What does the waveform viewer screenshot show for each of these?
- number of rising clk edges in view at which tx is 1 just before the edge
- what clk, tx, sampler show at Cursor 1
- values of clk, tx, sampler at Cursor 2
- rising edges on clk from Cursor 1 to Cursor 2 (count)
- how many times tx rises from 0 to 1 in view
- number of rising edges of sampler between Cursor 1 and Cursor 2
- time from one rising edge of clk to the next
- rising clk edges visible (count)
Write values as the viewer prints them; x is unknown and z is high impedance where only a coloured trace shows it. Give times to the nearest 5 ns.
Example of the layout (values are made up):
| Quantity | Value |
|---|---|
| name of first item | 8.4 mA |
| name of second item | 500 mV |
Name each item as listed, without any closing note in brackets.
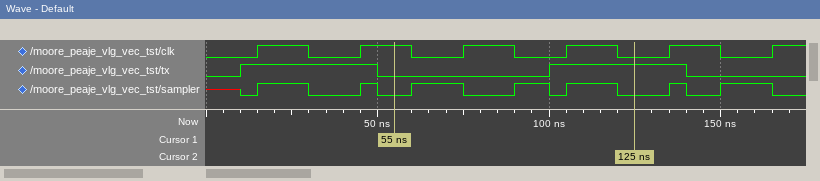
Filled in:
| Quantity | Value |
|---|---|
| number of rising clk edges in view at which tx is 1 just before the edge | 4 |
| what clk, tx, sampler show at Cursor 1 | clk=1, tx=0, sampler=0 |
| values of clk, tx, sampler at Cursor 2 | clk=0, tx=1, sampler=0 |
| rising edges on clk from Cursor 1 to Cursor 2 | 2 |
| how many times tx rises from 0 to 1 in view | 2 |
| number of rising edges of sampler between Cursor 1 and Cursor 2 | 3 |
| time from one rising edge of clk to the next | 30 ns |
| rising clk edges visible | 6 |
